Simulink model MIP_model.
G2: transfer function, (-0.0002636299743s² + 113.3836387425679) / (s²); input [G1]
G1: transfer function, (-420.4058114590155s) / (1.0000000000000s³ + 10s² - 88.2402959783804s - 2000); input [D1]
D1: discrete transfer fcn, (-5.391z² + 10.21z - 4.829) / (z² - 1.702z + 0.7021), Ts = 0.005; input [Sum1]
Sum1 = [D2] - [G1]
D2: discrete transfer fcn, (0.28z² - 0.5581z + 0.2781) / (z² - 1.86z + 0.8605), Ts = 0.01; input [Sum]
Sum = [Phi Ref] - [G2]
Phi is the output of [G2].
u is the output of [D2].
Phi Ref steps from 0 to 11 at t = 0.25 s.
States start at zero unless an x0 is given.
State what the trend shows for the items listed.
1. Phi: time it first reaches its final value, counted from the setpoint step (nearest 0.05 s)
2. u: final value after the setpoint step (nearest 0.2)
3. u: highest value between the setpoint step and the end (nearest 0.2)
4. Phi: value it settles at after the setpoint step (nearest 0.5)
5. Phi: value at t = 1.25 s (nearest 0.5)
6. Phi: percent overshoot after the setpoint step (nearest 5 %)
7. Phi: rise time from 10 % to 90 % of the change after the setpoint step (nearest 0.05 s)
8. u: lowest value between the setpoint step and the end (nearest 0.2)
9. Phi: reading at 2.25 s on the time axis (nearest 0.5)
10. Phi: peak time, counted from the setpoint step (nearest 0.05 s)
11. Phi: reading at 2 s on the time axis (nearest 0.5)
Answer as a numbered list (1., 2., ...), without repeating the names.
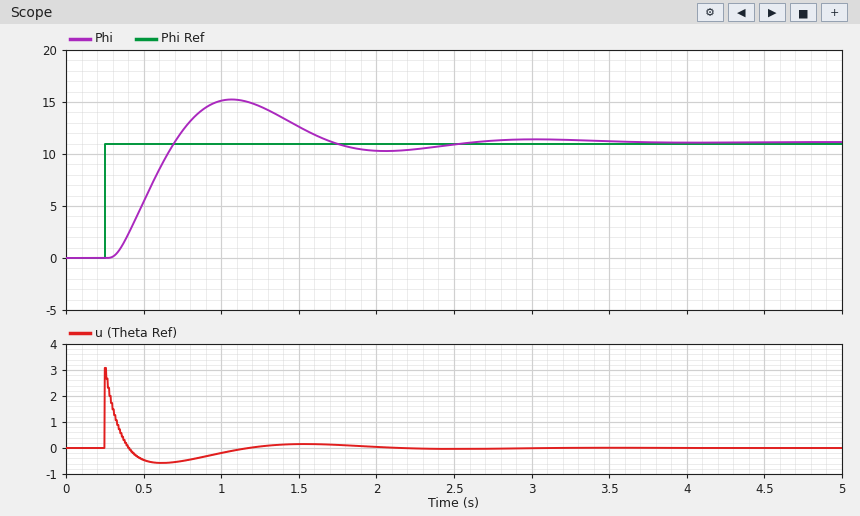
1. 0.45 s
2. 0.0
3. 3.0
4. 11.0
5. 14.5
6. 35 %
7. 0.30 s
8. -0.6
9. 10.5
10. 0.80 s
11. 10.5
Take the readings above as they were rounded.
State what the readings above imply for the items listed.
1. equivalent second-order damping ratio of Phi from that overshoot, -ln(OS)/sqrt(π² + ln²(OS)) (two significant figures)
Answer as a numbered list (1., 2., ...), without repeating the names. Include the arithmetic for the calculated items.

1. ln(0.35) = -1.050; 1.050 / sqrt(9.870 + 1.102) = 0.32
